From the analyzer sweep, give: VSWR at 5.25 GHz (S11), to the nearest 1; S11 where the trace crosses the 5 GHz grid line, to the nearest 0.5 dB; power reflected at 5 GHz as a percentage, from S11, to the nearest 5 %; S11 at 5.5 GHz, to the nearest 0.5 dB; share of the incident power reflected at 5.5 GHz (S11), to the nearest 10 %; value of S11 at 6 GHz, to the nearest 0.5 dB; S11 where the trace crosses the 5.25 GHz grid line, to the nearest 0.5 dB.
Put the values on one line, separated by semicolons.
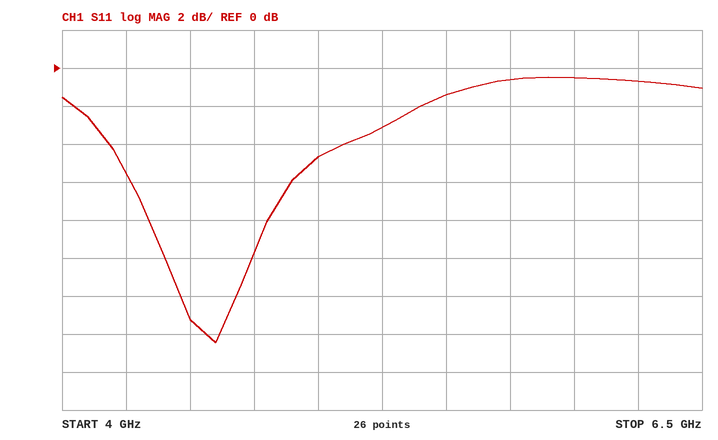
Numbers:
6; -4.5 dB; 35 %; -1.5 dB; 70 %; -0.5 dB; -3.0 dB
